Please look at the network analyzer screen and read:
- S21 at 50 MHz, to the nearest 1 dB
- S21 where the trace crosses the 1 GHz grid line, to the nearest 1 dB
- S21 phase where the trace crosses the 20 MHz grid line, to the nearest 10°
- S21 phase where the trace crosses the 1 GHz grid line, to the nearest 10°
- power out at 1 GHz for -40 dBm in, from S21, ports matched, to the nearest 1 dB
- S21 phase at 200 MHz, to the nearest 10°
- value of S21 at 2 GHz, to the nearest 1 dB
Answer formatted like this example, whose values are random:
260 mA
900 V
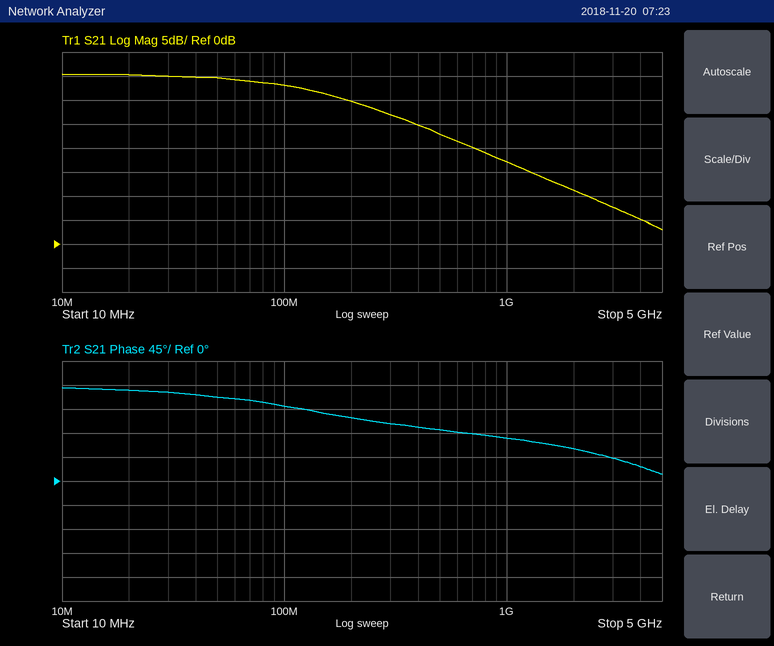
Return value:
35 dB
17 dB
170°
80°
-23 dBm
120°
11 dB
